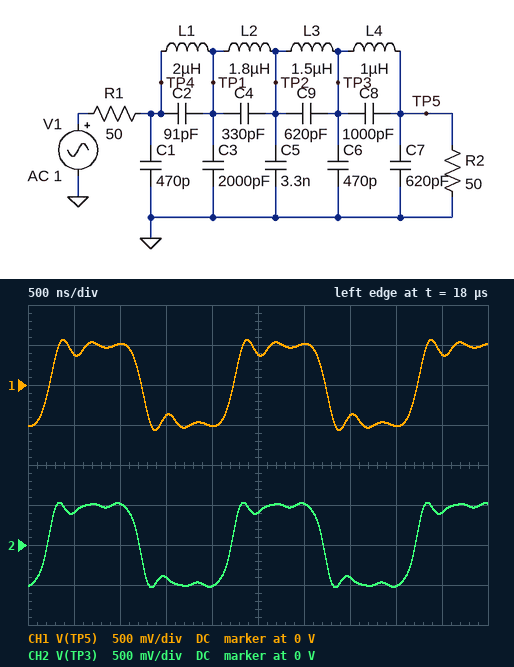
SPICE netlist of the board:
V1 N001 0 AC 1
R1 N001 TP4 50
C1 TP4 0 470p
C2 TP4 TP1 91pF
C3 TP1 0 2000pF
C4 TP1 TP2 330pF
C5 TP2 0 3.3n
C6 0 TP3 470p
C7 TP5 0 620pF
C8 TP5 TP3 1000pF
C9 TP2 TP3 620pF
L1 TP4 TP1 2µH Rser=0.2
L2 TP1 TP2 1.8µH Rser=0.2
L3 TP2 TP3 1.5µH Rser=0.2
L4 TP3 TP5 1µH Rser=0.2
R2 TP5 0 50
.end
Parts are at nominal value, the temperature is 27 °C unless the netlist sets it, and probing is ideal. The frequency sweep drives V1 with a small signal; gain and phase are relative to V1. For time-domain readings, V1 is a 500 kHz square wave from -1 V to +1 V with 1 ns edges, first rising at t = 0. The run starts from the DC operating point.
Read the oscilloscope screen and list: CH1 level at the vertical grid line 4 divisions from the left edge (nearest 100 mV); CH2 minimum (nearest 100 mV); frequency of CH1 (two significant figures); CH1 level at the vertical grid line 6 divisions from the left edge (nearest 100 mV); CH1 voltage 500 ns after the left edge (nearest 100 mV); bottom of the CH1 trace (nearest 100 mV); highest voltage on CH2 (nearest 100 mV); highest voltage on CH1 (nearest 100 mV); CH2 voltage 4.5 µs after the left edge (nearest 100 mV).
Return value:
-500 mV
-500 mV
500 kHz
500 mV
400 mV
-600 mV
500 mV
600 mV
400 mV
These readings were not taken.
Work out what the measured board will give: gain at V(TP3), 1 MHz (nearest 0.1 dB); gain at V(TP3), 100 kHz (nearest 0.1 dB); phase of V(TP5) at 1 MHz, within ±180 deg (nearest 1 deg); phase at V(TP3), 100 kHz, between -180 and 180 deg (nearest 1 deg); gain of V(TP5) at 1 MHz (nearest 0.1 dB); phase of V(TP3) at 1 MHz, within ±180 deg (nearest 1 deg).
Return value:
-7.4 dB
-6.1 dB
-79 deg
-8 deg
-7.3 dB
-71 deg
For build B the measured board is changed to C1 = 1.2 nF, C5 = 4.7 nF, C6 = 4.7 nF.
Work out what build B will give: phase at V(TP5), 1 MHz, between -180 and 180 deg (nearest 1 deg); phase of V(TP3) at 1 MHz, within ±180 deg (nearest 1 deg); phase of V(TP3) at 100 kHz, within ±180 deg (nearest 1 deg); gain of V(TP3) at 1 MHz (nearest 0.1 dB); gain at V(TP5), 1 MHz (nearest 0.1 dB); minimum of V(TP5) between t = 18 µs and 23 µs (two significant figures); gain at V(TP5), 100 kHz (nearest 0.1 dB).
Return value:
-103 deg
-95 deg
-13 deg
-9.4 dB
-9.3 dB
-490 mV
-6.2 dB
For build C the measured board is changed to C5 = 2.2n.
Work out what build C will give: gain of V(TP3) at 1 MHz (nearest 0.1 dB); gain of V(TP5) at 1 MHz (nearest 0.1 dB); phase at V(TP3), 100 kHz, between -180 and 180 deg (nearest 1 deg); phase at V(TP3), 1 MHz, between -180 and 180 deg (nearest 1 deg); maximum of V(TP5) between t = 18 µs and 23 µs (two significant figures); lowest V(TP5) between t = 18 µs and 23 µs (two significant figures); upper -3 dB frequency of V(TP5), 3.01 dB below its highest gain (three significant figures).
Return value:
-6.9 dB
-6.8 dB
-7 deg
-64 deg
640 mV
-640 mV
3.60 MHz
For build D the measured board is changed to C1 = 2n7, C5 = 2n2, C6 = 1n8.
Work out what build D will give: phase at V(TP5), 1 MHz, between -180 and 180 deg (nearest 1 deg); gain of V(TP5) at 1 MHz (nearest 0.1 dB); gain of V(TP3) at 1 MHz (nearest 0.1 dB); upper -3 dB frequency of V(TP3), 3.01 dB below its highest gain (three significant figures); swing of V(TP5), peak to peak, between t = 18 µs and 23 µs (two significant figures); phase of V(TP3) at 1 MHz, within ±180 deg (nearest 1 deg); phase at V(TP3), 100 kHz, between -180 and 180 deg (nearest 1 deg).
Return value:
-90 deg
-7.4 dB
-7.5 dB
3.95 MHz
1.2 V
-82 deg
-10 deg
